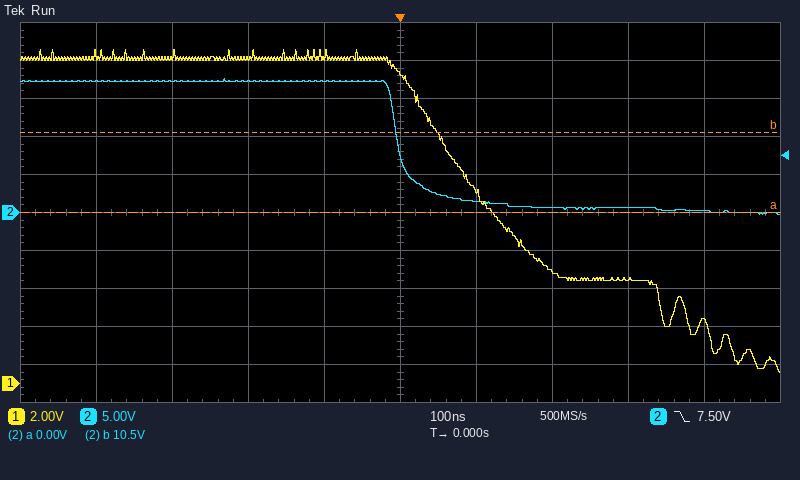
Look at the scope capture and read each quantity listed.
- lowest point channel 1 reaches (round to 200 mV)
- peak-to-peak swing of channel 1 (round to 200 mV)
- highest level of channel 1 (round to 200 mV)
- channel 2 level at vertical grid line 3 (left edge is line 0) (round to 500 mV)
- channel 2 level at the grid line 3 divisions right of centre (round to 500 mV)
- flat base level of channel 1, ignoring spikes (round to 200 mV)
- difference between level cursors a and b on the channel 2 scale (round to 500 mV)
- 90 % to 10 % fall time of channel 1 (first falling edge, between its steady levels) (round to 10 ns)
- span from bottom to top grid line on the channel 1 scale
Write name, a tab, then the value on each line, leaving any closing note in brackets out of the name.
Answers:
lowest point channel 1 reaches	600 mV
peak-to-peak swing of channel 1	17.0 V
highest level of channel 1	17.6 V
channel 2 level at vertical grid line 3 (left edge is line 0)	17.5 V
channel 2 level at the grid line 3 divisions right of centre	500 mV
flat base level of channel 1, ignoring spikes	5.4 V
difference between level cursors a and b on the channel 2 scale	10.5 V
90 % to 10 % fall time of channel 1 (first falling edge, between its steady levels)	170 ns
span from bottom to top grid line on the channel 1 scale	20 V
